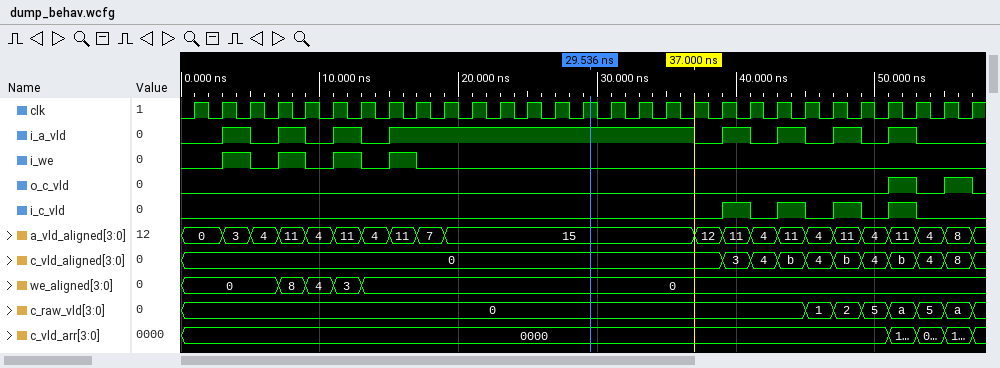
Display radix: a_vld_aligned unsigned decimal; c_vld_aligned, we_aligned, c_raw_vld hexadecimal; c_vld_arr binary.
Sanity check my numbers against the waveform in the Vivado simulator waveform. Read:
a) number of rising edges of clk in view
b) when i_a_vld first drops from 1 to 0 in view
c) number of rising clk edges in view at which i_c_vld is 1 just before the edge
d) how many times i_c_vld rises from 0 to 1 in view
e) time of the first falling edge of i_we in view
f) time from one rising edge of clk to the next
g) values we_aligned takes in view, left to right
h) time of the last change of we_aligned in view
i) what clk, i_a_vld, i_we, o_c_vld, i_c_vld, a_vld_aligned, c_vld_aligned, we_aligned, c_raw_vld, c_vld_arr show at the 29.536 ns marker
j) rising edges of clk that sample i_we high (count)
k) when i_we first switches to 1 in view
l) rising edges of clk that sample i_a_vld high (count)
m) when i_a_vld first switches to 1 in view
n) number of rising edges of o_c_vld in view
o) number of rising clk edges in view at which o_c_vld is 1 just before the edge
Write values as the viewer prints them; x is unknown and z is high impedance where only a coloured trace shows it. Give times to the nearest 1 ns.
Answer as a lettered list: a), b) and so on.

a) 29
b) 5 ns
c) 4
d) 4
e) 5 ns
f) 2 ns
g) 0, 8, 4, 3, 0
h) 13 ns
i) clk=1, i_a_vld=1, i_we=0, o_c_vld=0, i_c_vld=0, a_vld_aligned=15, c_vld_aligned=0, we_aligned=0, c_raw_vld=0, c_vld_arr=0000
j) 4
k) 3 ns
l) 18
m) 3 ns
n) 2
o) 2
